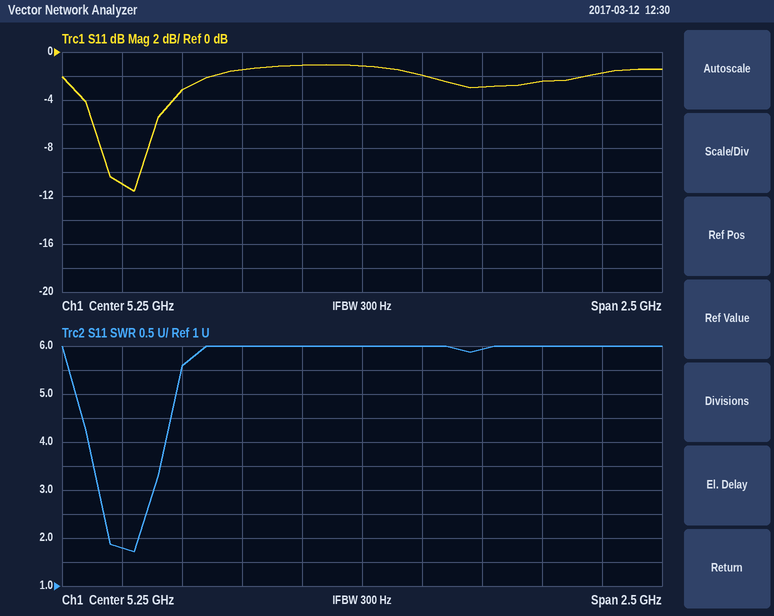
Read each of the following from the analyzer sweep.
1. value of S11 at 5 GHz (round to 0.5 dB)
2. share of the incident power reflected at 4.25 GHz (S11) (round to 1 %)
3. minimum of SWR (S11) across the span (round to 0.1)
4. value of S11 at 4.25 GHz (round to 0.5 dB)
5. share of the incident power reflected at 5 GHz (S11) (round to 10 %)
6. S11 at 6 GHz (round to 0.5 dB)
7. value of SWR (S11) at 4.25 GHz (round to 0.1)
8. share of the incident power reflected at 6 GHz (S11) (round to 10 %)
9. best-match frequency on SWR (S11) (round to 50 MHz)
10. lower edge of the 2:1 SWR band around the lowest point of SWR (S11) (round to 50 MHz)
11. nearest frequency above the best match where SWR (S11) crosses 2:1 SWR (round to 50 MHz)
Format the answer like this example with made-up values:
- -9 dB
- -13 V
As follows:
- -1.0 dB
- 8 %
- 1.7
- -11.0 dB
- 80 %
- -2.5 dB
- 1.8
- 60 %
- 4.30 GHz
- 4.20 GHz
- 4.30 GHz
